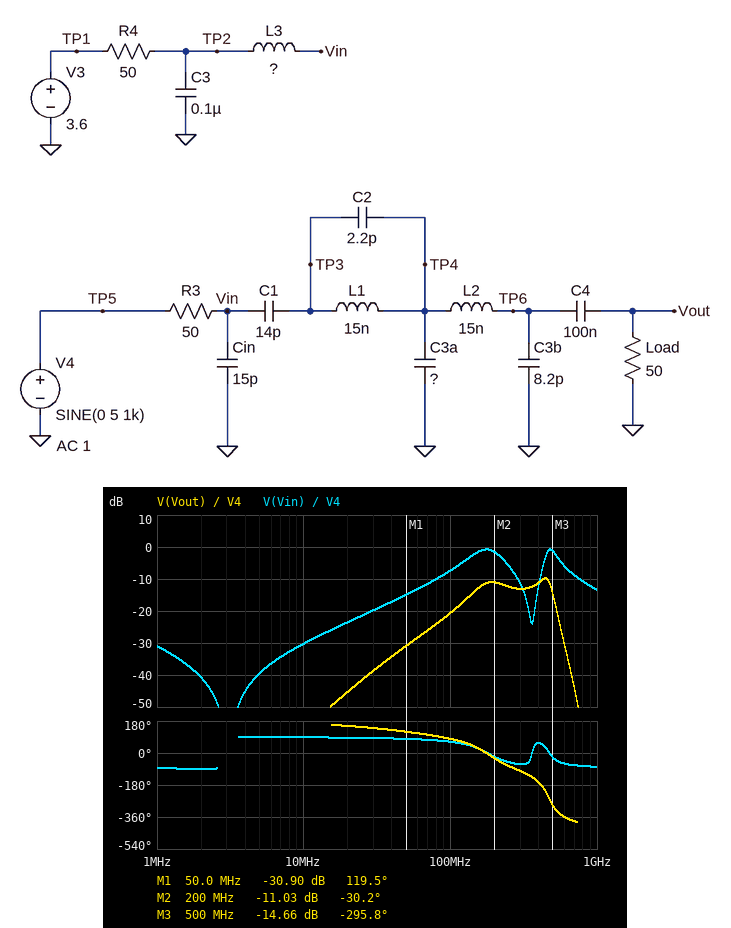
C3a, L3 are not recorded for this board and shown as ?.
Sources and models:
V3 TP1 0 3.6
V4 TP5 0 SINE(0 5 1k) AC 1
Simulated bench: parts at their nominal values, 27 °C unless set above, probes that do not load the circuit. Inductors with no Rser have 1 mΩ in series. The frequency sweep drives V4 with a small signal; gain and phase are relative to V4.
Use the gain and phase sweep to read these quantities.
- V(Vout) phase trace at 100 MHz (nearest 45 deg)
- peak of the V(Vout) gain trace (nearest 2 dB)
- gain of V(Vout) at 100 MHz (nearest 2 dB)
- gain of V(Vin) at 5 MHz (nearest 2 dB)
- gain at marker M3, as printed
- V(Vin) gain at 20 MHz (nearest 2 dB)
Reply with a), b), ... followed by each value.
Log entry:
a) 90 deg
b) -10 dB
c) -20 dB
d) -40 dB
e) -14.66 dB
f) -24 dB
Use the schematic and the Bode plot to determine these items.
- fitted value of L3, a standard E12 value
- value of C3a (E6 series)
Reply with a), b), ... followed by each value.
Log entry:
a) 27 nH
b) 47 pF
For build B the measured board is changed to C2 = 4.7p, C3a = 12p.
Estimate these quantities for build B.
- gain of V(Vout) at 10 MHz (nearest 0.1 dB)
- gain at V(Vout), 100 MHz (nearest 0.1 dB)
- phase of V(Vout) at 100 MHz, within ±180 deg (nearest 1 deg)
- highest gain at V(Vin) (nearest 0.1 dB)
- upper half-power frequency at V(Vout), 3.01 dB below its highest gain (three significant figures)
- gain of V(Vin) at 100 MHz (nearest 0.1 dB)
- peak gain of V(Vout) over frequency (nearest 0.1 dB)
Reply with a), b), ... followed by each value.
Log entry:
a) -57.4 dB
b) -16.6 dB
c) 100 deg
d) -2.4 dB
e) 456 MHz
f) -7.6 dB
g) -6.0 dB
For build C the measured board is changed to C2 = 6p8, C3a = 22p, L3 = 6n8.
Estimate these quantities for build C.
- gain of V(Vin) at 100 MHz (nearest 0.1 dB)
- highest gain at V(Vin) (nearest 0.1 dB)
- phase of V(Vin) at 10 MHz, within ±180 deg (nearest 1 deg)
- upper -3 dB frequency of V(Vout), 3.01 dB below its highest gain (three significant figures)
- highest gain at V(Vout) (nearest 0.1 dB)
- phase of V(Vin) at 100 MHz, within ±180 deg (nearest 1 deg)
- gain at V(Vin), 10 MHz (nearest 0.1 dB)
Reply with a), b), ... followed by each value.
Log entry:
a) -20.8 dB
b) 0 dB
c) 89 deg
d) 331 MHz
e) -6.7 dB
f) 84 deg
g) -45.4 dB
